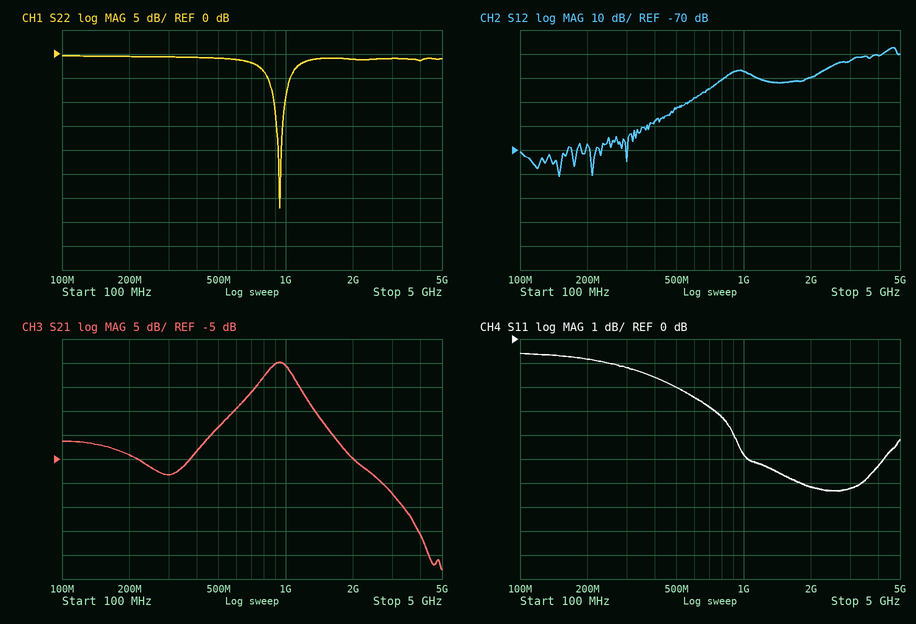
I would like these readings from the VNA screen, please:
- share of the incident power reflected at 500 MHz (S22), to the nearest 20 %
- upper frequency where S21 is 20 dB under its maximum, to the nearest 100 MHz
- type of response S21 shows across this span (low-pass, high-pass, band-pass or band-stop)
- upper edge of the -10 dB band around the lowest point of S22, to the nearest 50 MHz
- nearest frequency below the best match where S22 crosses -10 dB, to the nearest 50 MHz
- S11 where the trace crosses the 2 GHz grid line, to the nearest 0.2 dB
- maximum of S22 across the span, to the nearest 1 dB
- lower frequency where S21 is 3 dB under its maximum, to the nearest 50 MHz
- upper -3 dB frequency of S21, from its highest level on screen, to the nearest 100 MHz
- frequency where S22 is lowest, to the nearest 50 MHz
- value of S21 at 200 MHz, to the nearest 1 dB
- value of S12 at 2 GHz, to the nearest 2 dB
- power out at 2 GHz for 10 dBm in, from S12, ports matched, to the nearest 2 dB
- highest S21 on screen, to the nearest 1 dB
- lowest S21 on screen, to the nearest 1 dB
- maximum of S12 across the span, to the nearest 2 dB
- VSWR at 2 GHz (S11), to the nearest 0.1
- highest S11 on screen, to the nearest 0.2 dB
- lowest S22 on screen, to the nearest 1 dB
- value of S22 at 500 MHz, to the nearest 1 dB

80 %
2.0 GHz
band-pass
1.00 GHz
900 MHz
-6.2 dB
0 dB
800 MHz
1.1 GHz
950 MHz
-4 dB
-40 dB
-30 dBm
15 dB
-28 dB
-28 dB
2.9
-0.6 dB
-32 dB
-1 dB
